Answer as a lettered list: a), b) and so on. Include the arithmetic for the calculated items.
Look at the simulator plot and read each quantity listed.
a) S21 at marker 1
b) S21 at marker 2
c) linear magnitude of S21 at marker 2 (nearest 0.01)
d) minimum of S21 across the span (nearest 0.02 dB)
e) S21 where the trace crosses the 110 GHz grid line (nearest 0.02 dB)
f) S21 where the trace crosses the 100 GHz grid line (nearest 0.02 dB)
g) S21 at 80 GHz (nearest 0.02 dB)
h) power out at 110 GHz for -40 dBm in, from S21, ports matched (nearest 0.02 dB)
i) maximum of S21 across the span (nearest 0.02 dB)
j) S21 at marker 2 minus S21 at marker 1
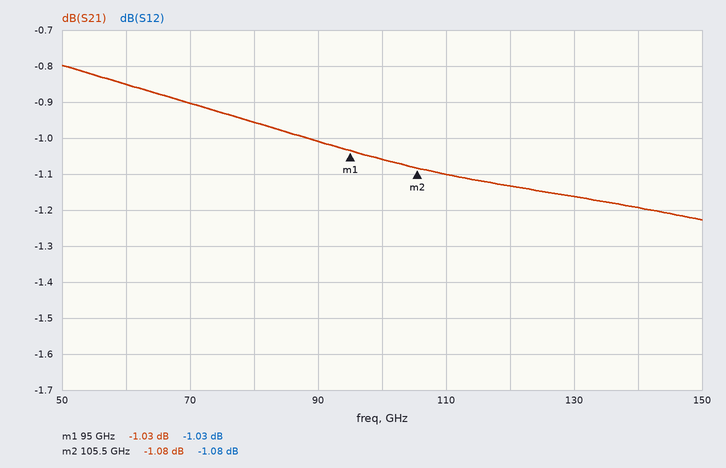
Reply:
a) -1.03 dB
b) -1.08 dB
c) 10^(-1.08/20) ≈ 0.88
d) -1.22 dB
e) -1.10 dB
f) -1.06 dB
g) -0.96 dB
h) -40 dBm + (-1.10 dB) = -41.10 dBm
i) -0.80 dB
j) -1.08 − (-1.03) = -0.05 dB
